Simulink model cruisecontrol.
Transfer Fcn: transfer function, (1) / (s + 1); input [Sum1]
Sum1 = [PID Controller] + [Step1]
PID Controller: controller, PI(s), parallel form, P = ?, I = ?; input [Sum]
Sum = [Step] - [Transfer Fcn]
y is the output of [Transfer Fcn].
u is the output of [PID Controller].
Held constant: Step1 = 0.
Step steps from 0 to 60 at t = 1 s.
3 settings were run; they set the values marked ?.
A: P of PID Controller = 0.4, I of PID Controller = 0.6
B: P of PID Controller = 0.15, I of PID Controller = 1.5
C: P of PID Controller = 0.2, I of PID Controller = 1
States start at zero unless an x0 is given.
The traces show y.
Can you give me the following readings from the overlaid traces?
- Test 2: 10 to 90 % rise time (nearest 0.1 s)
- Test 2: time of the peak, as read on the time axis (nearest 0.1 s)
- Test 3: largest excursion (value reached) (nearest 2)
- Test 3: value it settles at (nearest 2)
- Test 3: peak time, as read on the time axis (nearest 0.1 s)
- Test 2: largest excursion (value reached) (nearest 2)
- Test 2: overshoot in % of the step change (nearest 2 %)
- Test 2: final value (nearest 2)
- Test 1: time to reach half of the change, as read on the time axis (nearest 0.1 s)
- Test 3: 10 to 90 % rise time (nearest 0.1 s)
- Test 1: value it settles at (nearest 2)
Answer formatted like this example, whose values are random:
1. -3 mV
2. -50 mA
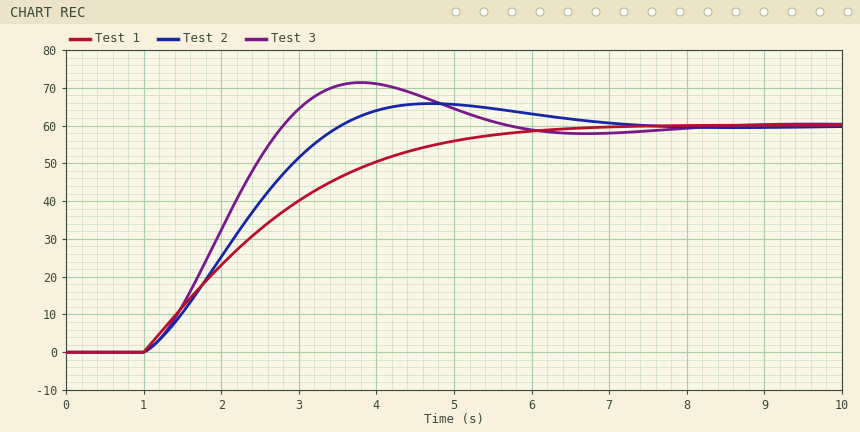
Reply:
1. 1.8 s
2. 4.7 s
3. 72
4. 60
5. 3.8 s
6. 66
7. 10 %
8. 60
9. 2.4 s
10. 1.3 s
11. 60
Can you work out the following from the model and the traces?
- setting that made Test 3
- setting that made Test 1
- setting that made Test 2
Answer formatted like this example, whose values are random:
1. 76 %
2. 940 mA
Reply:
1. B
2. A
3. C
